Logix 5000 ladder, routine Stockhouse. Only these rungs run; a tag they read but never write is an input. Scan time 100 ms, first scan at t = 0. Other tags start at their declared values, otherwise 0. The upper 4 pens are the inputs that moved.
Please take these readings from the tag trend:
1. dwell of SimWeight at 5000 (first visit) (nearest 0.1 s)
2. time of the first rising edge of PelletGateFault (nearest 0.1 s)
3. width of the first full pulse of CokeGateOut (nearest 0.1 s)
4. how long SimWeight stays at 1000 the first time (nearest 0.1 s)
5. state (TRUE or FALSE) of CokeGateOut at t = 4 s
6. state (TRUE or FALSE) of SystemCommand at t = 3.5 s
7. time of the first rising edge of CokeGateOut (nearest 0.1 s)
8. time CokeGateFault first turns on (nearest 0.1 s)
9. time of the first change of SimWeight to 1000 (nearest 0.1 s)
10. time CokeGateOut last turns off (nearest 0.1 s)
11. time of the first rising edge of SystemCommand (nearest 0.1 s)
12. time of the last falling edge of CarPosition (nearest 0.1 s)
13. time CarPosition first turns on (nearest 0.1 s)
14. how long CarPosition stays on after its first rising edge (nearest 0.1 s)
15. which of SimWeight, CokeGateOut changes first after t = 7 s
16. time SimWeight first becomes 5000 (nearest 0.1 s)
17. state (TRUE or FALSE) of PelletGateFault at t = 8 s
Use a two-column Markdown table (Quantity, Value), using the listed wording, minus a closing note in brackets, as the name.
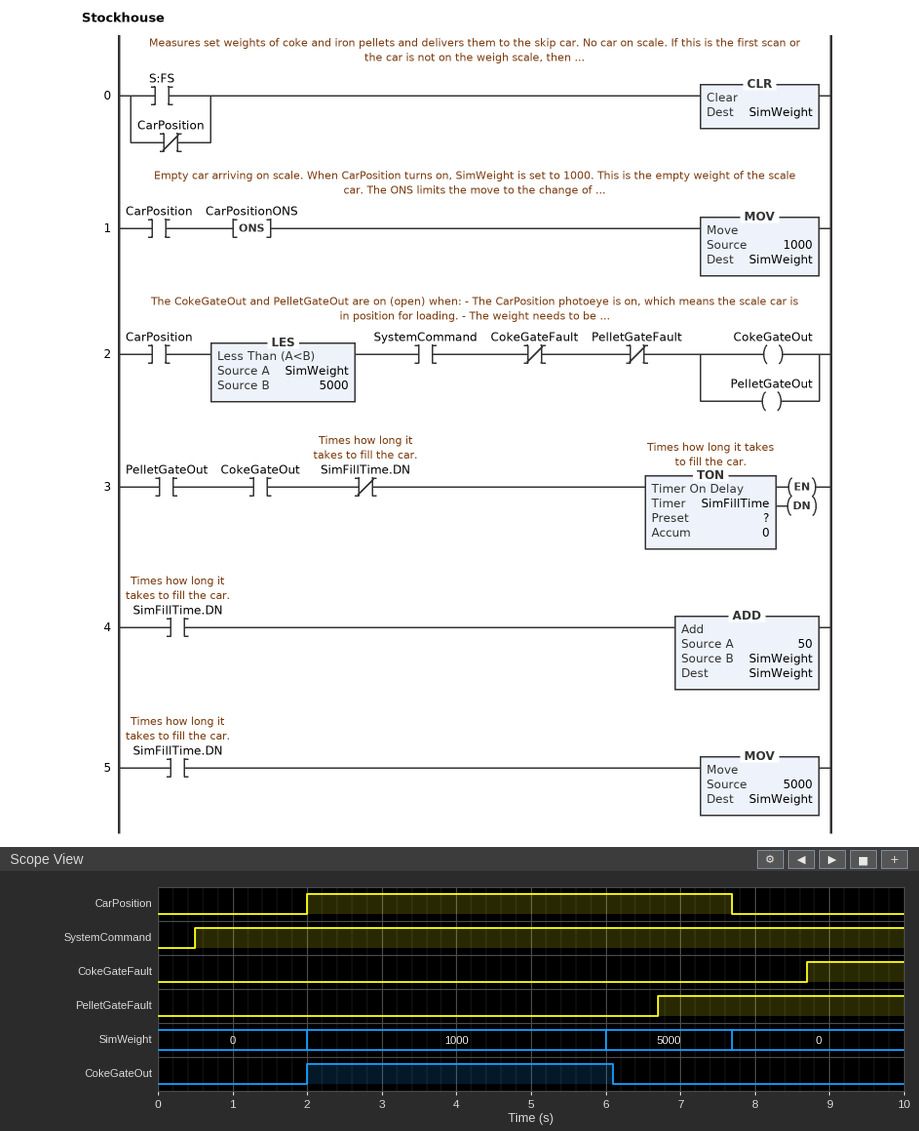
| Quantity | Value |
|---|---|
| dwell of SimWeight at 5000 (first visit) | 1.7 s |
| time of the first rising edge of PelletGateFault | 6.7 s |
| width of the first full pulse of CokeGateOut | 4.1 s |
| how long SimWeight stays at 1000 the first time | 4.0 s |
| state (TRUE or FALSE) of CokeGateOut at t = 4 s | TRUE |
| state (TRUE or FALSE) of SystemCommand at t = 3.5 s | TRUE |
| time of the first rising edge of CokeGateOut | 2.0 s |
| time CokeGateFault first turns on | 8.7 s |
| time of the first change of SimWeight to 1000 | 2.0 s |
| time CokeGateOut last turns off | 6.1 s |
| time of the first rising edge of SystemCommand | 0.5 s |
| time of the last falling edge of CarPosition | 7.7 s |
| time CarPosition first turns on | 2.0 s |
| how long CarPosition stays on after its first rising edge | 5.7 s |
| which of SimWeight, CokeGateOut changes first after t = 7 s | SimWeight |
| time SimWeight first becomes 5000 | 6.0 s |
| state (TRUE or FALSE) of PelletGateFault at t = 8 s | TRUE |
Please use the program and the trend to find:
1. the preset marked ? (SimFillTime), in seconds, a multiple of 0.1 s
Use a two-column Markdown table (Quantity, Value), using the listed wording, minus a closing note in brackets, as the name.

| Quantity | Value |
|---|---|
| the preset marked ? (SimFillTime), in seconds, a multiple of 0.1 s | 4.0 s |
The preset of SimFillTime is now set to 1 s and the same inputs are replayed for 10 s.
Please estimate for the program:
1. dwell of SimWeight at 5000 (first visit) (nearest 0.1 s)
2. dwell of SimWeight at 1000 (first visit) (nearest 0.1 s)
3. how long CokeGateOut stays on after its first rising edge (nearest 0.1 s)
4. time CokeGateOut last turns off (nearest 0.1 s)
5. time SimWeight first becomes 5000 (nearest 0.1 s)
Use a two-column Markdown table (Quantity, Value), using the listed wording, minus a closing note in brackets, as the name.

| Quantity | Value |
|---|---|
| dwell of SimWeight at 5000 (first visit) | 4.7 s |
| dwell of SimWeight at 1000 (first visit) | 1.0 s |
| how long CokeGateOut stays on after its first rising edge | 1.1 s |
| time CokeGateOut last turns off | 3.1 s |
| time SimWeight first becomes 5000 | 3.0 s |
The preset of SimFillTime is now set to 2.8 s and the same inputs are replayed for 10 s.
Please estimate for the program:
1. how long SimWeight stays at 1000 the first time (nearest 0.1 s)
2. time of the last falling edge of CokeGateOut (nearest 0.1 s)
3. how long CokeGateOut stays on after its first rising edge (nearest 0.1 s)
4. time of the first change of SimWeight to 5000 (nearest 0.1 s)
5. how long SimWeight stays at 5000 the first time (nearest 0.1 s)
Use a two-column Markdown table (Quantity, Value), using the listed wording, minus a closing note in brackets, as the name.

| Quantity | Value |
|---|---|
| how long SimWeight stays at 1000 the first time | 2.8 s |
| time of the last falling edge of CokeGateOut | 4.9 s |
| how long CokeGateOut stays on after its first rising edge | 2.9 s |
| time of the first change of SimWeight to 5000 | 4.8 s |
| how long SimWeight stays at 5000 the first time | 2.9 s |
